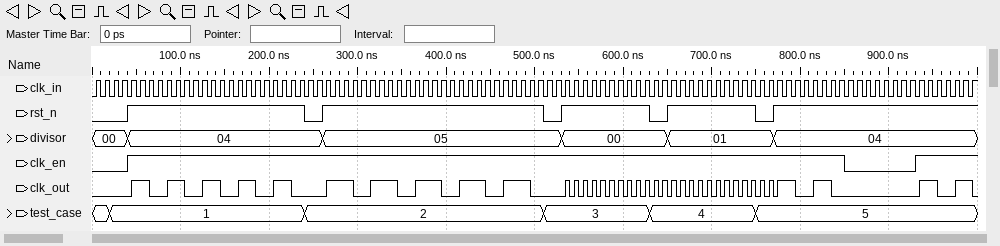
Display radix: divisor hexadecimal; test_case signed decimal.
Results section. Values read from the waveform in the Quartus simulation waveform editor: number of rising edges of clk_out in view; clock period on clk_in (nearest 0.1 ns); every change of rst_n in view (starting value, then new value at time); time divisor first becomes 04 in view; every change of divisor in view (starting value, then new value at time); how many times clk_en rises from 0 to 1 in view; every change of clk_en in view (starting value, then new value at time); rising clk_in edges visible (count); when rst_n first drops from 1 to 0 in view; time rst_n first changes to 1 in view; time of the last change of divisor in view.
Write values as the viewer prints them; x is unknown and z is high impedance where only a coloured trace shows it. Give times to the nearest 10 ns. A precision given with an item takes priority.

38
10 ns
0, 1 at 40 ns, 0 at 240 ns, 1 at 260 ns, 0 at 510 ns, 1 at 530 ns, 0 at 630 ns, 1 at 650 ns, 0 at 750 ns, 1 at 770 ns
40 ns
00, 04 at 40 ns, 05 at 260 ns, 00 at 530 ns, 01 at 650 ns, 04 at 770 ns
2
0, 1 at 40 ns, 0 at 850 ns, 1 at 930 ns
100
240 ns
40 ns
770 ns
